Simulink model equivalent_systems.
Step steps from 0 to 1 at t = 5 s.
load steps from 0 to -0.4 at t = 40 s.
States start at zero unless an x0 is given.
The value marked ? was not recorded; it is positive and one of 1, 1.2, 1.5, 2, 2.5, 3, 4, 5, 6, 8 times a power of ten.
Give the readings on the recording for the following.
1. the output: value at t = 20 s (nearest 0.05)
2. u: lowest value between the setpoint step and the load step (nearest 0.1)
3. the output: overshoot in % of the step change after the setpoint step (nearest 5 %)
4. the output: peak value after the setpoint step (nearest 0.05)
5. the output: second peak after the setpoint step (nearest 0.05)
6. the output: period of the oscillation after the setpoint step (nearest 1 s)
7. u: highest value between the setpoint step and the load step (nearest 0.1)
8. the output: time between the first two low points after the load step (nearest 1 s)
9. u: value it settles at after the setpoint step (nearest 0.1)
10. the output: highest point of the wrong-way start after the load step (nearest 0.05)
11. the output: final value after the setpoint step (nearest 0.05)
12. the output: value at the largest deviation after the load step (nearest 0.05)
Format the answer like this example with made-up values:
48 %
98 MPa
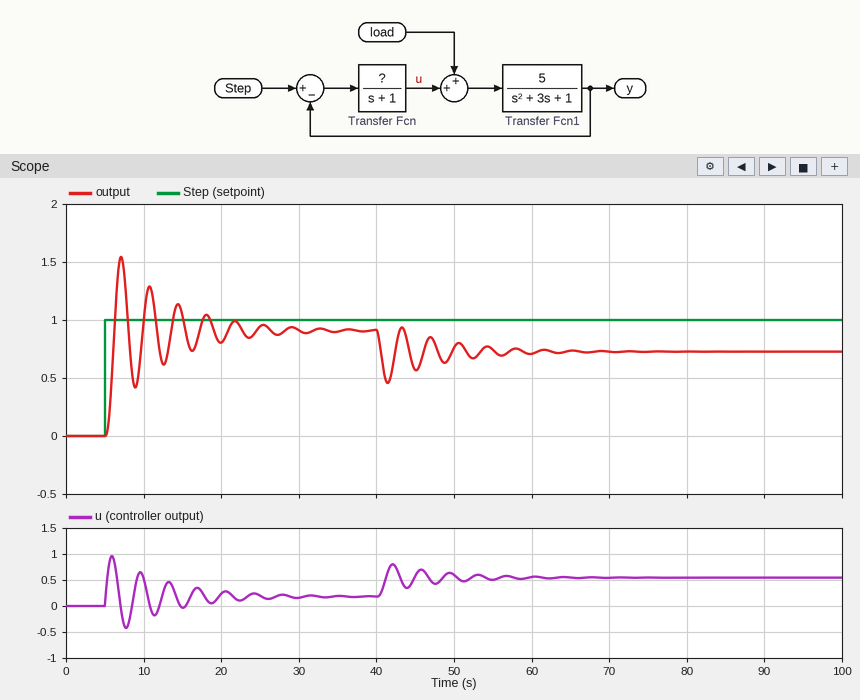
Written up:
0.80
-0.4
70 %
1.55
1.30
4 s
1.0
4 s
0.2
0.95
0.90
0.45
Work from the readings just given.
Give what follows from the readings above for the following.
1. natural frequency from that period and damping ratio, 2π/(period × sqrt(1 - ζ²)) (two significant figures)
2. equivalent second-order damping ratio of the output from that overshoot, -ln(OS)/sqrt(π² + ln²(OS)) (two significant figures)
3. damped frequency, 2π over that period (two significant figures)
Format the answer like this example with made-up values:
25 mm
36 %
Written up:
1.6 rad/s
0.11
1.6 rad/s
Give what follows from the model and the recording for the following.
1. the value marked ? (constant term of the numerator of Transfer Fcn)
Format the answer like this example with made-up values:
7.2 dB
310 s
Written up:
2
